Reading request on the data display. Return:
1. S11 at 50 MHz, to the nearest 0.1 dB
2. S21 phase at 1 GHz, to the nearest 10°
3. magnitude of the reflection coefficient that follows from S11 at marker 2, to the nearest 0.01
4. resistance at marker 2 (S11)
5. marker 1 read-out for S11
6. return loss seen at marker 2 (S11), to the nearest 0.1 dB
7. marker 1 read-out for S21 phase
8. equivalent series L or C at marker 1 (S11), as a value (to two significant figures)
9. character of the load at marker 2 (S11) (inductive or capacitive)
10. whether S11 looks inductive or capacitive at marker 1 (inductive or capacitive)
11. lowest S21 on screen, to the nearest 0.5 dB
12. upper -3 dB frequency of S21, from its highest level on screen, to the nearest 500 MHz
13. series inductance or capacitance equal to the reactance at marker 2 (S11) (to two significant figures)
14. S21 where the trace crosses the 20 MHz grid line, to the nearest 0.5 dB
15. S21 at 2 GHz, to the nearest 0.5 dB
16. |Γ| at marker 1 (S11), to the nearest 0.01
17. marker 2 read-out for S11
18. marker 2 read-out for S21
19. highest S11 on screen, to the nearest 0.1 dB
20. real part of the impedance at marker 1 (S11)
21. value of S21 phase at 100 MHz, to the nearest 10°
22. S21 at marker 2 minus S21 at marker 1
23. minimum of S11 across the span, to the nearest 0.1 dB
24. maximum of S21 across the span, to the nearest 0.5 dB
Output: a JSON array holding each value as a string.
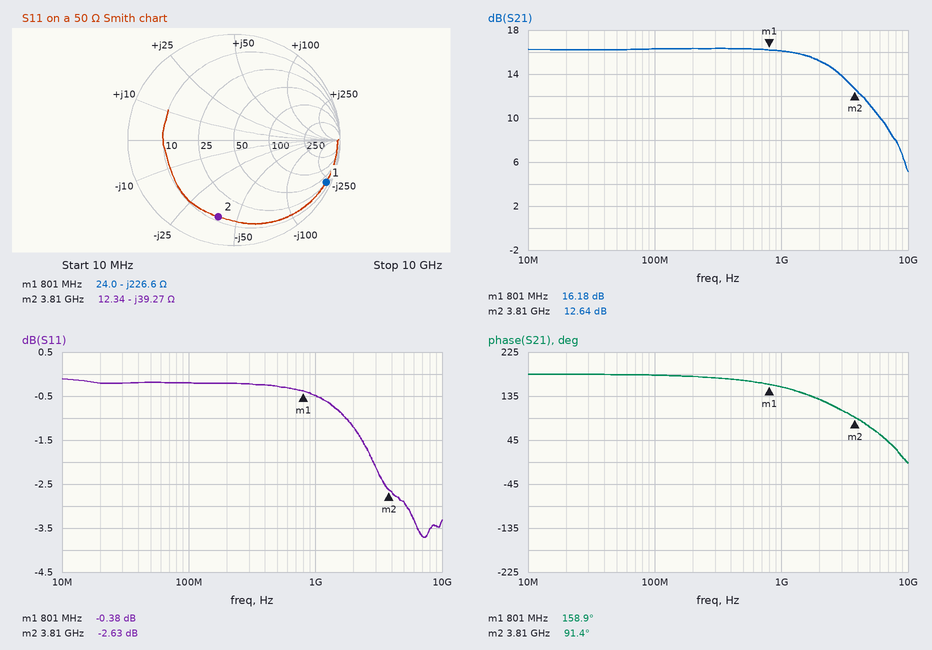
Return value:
["-0.2 dB", "150°", "0.74", "12.34 Ω", "-0.38 dB", "2.6 dB", "158.9°", "880 fF", "capacitive", "capacitive", "5.0 dB", "3.5 GHz", "1.1 pF", "16.0 dB", "15.0 dB", "0.96", "-2.63 dB", "12.64 dB", "-0.1 dB", "24.0 Ω", "180°", "-3.54 dB", "-3.7 dB", "16.5 dB"]
